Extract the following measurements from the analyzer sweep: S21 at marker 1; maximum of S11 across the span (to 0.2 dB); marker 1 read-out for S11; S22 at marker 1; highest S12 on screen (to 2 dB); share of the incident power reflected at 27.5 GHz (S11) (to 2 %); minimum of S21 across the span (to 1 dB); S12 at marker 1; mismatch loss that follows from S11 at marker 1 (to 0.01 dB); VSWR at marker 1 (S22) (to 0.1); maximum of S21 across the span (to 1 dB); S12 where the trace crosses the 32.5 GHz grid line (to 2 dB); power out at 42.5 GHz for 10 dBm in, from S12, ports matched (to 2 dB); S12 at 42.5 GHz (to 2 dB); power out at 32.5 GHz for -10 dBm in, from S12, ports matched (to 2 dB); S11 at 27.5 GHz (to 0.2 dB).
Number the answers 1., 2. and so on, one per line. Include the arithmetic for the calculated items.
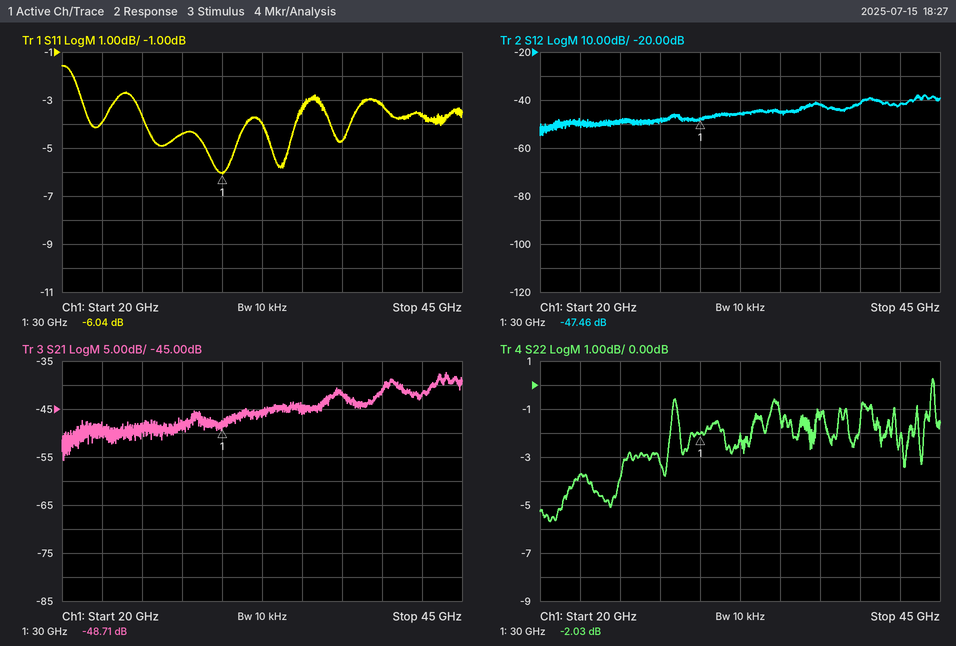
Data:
1. -48.71 dB
2. -1.6 dB
3. -6.04 dB
4. -2.03 dB
5. -38 dB
6. 10^(-4.4/10) ≈ 36 %
7. -56 dB
8. -47.46 dB
9. −10 log10(1 − 10^(-6.04/10)) ≈ 1.24 dB
10. (1 + 0.7916)/(1 − 0.7916) ≈ 8.6
11. -37 dB
12. -46 dB
13. 10 dBm + (-42 dB) = -32 dBm
14. -42 dB
15. -10 dBm + (-46 dB) = -56 dBm
16. -4.4 dB
